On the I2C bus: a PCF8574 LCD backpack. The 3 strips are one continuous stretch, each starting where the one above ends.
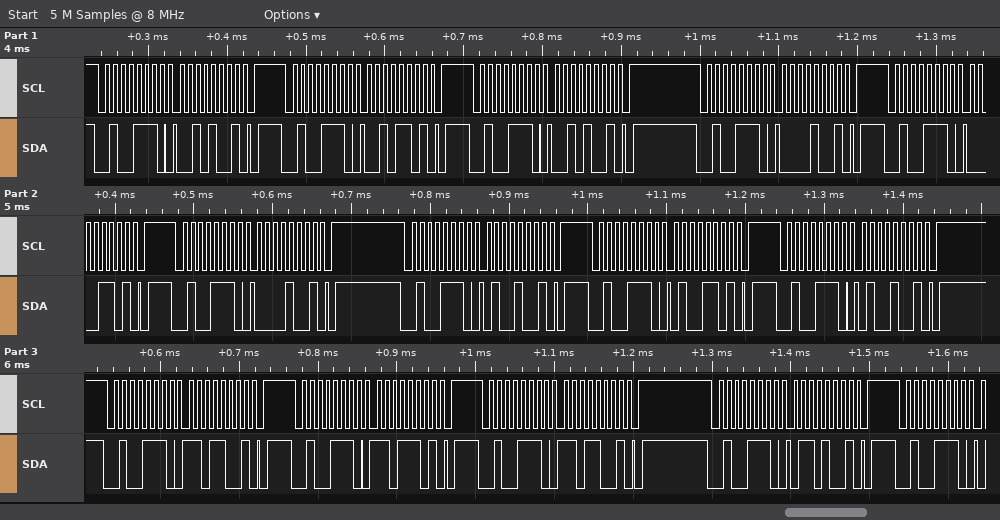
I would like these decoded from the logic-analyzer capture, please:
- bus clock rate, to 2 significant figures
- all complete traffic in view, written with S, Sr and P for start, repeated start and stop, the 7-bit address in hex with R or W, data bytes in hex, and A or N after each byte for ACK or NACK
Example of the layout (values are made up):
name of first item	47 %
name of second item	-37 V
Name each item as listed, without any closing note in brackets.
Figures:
bus clock rate, to 2 significant figures	100 kHz
all complete traffic in view, written with S, Sr and P for start, repeated start and stop, the 7-bit address in hex with R or W, data bytes in hex, and A or N after each byte for ACK or NACK	S 27W A 29 A P S 27W A 2D A P S 27W A 29 A P S 27W A 09 A P S 27W A 0D A P S 27W A 09 A P S 27W A 49 A P S 27W A 4D A P S 27W A 49 A P S 27W A D9 A P S 27W A DD A P S 27W A D9 A P S 27W A 69 A P S 27W A
